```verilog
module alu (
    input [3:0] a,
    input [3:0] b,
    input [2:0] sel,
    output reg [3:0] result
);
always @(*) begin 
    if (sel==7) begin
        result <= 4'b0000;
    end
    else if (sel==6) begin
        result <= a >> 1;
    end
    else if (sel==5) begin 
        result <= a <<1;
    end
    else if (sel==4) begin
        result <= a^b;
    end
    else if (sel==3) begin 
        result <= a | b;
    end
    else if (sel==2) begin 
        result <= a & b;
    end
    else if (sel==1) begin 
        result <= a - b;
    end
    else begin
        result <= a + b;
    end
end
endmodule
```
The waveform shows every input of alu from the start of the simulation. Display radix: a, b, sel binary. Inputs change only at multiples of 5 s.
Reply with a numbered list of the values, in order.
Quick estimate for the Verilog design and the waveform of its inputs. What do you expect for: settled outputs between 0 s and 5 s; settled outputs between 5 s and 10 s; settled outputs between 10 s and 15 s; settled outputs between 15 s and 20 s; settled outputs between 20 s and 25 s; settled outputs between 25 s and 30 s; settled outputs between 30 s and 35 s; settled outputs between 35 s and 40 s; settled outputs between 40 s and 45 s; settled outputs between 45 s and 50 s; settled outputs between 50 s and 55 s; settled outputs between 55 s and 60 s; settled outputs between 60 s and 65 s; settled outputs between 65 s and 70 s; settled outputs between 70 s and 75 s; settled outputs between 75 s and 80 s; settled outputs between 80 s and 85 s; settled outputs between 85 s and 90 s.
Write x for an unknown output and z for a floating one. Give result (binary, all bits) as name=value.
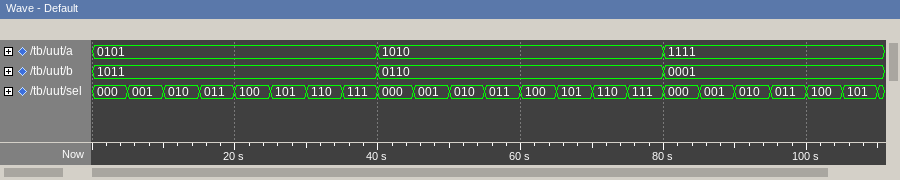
1. result=0000
2. result=1010
3. result=0001
4. result=1111
5. result=1110
6. result=1010
7. result=0010
8. result=0000
9. result=0000
10. result=0100
11. result=0010
12. result=1110
13. result=1100
14. result=0100
15. result=0101
16. result=0000
17. result=0000
18. result=1110
